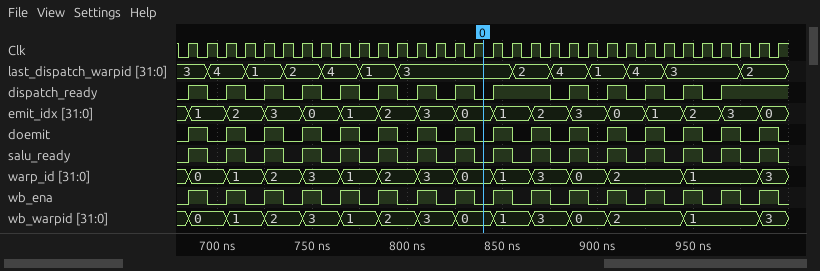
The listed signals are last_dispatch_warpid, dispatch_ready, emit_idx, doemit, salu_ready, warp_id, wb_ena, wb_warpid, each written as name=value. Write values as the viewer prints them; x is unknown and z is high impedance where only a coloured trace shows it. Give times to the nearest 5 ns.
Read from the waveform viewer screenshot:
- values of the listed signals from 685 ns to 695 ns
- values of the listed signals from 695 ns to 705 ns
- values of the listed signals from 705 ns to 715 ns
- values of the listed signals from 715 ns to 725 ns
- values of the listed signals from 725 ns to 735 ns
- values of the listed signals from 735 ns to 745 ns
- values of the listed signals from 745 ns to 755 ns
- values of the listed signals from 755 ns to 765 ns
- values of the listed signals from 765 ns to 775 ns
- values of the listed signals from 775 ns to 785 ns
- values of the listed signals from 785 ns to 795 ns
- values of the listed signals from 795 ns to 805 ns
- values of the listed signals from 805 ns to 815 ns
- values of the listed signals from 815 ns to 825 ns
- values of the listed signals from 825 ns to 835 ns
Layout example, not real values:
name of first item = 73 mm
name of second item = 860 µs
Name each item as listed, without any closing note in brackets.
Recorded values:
values of the listed signals from 685 ns to 695 ns = last_dispatch_warpid=3, dispatch_ready=1, emit_idx=1, doemit=1, salu_ready=1, warp_id=0, wb_ena=1, wb_warpid=0
values of the listed signals from 695 ns to 705 ns = last_dispatch_warpid=4, dispatch_ready=0, emit_idx=1, doemit=0, salu_ready=0, warp_id=0, wb_ena=0, wb_warpid=0
values of the listed signals from 705 ns to 715 ns = last_dispatch_warpid=4, dispatch_ready=1, emit_idx=2, doemit=1, salu_ready=1, warp_id=1, wb_ena=1, wb_warpid=1
values of the listed signals from 715 ns to 725 ns = last_dispatch_warpid=1, dispatch_ready=0, emit_idx=2, doemit=0, salu_ready=0, warp_id=1, wb_ena=0, wb_warpid=1
values of the listed signals from 725 ns to 735 ns = last_dispatch_warpid=1, dispatch_ready=1, emit_idx=3, doemit=1, salu_ready=1, warp_id=2, wb_ena=1, wb_warpid=2
values of the listed signals from 735 ns to 745 ns = last_dispatch_warpid=2, dispatch_ready=0, emit_idx=3, doemit=0, salu_ready=0, warp_id=2, wb_ena=0, wb_warpid=2
values of the listed signals from 745 ns to 755 ns = last_dispatch_warpid=2, dispatch_ready=1, emit_idx=0, doemit=1, salu_ready=1, warp_id=3, wb_ena=1, wb_warpid=3
values of the listed signals from 755 ns to 765 ns = last_dispatch_warpid=4, dispatch_ready=0, emit_idx=0, doemit=0, salu_ready=0, warp_id=3, wb_ena=0, wb_warpid=3
values of the listed signals from 765 ns to 775 ns = last_dispatch_warpid=4, dispatch_ready=1, emit_idx=1, doemit=1, salu_ready=1, warp_id=1, wb_ena=1, wb_warpid=1
values of the listed signals from 775 ns to 785 ns = last_dispatch_warpid=1, dispatch_ready=0, emit_idx=1, doemit=0, salu_ready=0, warp_id=1, wb_ena=0, wb_warpid=1
values of the listed signals from 785 ns to 795 ns = last_dispatch_warpid=1, dispatch_ready=1, emit_idx=2, doemit=1, salu_ready=1, warp_id=2, wb_ena=1, wb_warpid=2
values of the listed signals from 795 ns to 805 ns = last_dispatch_warpid=3, dispatch_ready=0, emit_idx=2, doemit=0, salu_ready=0, warp_id=2, wb_ena=0, wb_warpid=2
values of the listed signals from 805 ns to 815 ns = last_dispatch_warpid=3, dispatch_ready=1, emit_idx=3, doemit=1, salu_ready=1, warp_id=3, wb_ena=1, wb_warpid=3
values of the listed signals from 815 ns to 825 ns = last_dispatch_warpid=3, dispatch_ready=0, emit_idx=3, doemit=0, salu_ready=0, warp_id=3, wb_ena=0, wb_warpid=3
values of the listed signals from 825 ns to 835 ns = last_dispatch_warpid=3, dispatch_ready=1, emit_idx=0, doemit=1, salu_ready=1, warp_id=0, wb_ena=1, wb_warpid=0
